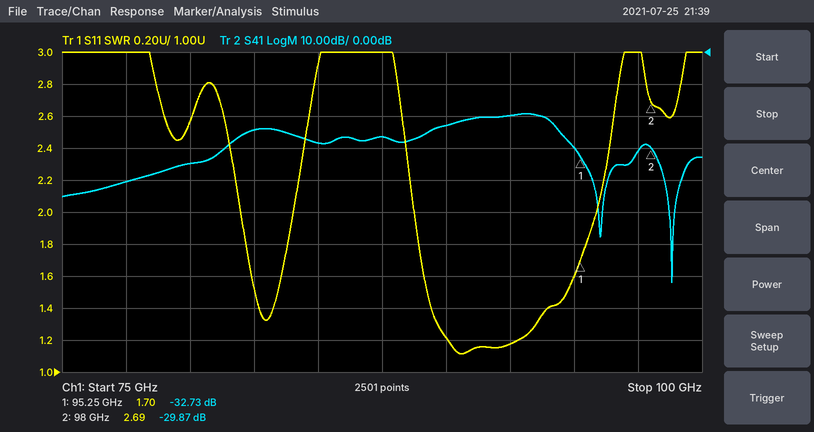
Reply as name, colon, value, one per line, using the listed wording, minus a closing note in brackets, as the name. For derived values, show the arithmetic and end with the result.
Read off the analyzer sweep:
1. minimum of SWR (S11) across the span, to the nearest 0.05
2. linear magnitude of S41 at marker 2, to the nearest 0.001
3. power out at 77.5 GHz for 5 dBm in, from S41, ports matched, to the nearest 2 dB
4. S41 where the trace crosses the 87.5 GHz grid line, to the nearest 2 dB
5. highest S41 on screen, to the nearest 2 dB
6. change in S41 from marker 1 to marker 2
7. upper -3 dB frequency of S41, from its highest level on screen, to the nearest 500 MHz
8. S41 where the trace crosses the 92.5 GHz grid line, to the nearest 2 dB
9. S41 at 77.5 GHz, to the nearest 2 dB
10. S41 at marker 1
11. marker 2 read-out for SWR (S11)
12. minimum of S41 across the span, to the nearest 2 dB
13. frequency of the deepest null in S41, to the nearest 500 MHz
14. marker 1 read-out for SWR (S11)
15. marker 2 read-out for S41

minimum of SWR (S11) across the span, to the nearest 0.05: 1.10
linear magnitude of S41 at marker 2, to the nearest 0.001: 10^(-29.87/20) ≈ 0.032
power out at 77.5 GHz for 5 dBm in, from S41, ports matched, to the nearest 2 dB: 5 dBm + (-40 dB) = -36 dBm
S41 where the trace crosses the 87.5 GHz grid line, to the nearest 2 dB: -26 dB
highest S41 on screen, to the nearest 2 dB: -20 dB
change in S41 from marker 1 to marker 2: -29.87 − (-32.73) = 2.86 dB
upper -3 dB frequency of S41, from its highest level on screen, to the nearest 500 MHz: 94.0 GHz
S41 where the trace crosses the 92.5 GHz grid line, to the nearest 2 dB: -20 dB
S41 at 77.5 GHz, to the nearest 2 dB: -40 dB
S41 at marker 1: -32.73 dB
marker 2 read-out for SWR: 2.69
minimum of S41 across the span, to the nearest 2 dB: -72 dB
frequency of the deepest null in S41, to the nearest 500 MHz: 99.0 GHz
marker 1 read-out for SWR: 1.70
marker 2 read-out for S41: -29.87 dB
